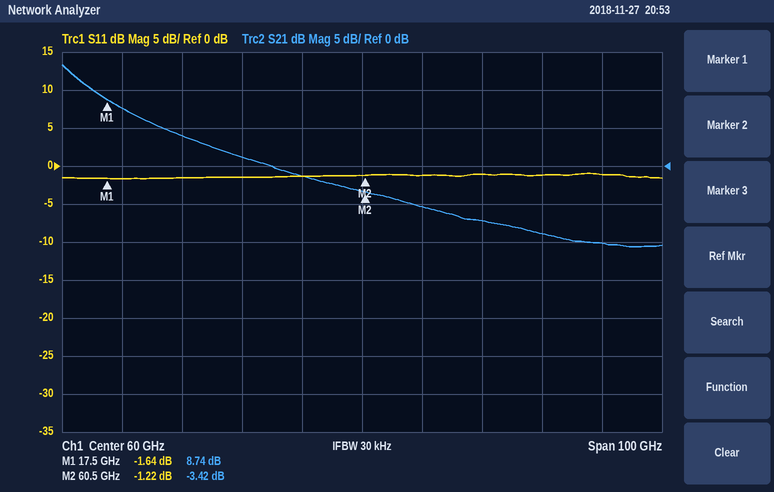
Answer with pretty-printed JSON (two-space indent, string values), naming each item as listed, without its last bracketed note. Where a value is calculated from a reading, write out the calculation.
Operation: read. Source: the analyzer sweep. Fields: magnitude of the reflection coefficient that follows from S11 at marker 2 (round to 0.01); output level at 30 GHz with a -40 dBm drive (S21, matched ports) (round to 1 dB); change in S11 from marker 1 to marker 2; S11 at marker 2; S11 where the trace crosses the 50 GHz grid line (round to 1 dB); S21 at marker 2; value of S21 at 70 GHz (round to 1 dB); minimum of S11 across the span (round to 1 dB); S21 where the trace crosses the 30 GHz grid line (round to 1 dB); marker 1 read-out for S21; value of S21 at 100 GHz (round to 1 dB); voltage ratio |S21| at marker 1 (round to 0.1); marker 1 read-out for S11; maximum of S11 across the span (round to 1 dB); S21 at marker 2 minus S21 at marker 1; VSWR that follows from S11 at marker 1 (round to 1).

{
  "magnitude of the reflection coefficient that follows from S11 at marker 2": "10^(-1.22/20) ≈ 0.87",
  "output level at 30 GHz with a -40 dBm drive (S21, matched ports)": "-40 dBm + (4 dB) = -36 dBm",
  "change in S11 from marker 1 to marker 2": "-1.22 − (-1.64) = 0.42 dB",
  "S11 at marker 2": "-1.22 dB",
  "S11 where the trace crosses the 50 GHz grid line": "-1 dB",
  "S21 at marker 2": "-3.42 dB",
  "value of S21 at 70 GHz": "-5 dB",
  "minimum of S11 across the span": "-2 dB",
  "S21 where the trace crosses the 30 GHz grid line": "4 dB",
  "marker 1 read-out for S21": "8.74 dB",
  "value of S21 at 100 GHz": "-10 dB",
  "voltage ratio |S21| at marker 1": "10^(8.74/20) ≈ 2.7",
  "marker 1 read-out for S11": "-1.64 dB",
  "maximum of S11 across the span": "-1 dB",
  "S21 at marker 2 minus S21 at marker 1": "-3.42 − (8.74) = -12.16 dB",
  "VSWR that follows from S11 at marker 1": "(1 + 0.8279)/(1 − 0.8279) ≈ 11"
}
